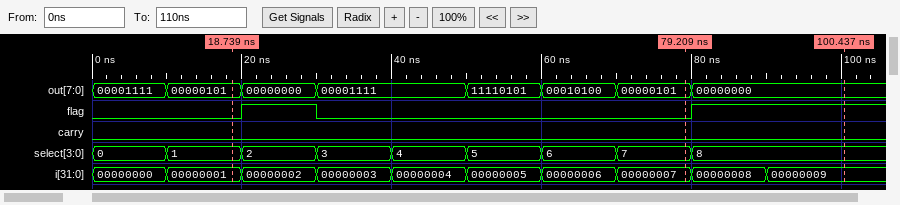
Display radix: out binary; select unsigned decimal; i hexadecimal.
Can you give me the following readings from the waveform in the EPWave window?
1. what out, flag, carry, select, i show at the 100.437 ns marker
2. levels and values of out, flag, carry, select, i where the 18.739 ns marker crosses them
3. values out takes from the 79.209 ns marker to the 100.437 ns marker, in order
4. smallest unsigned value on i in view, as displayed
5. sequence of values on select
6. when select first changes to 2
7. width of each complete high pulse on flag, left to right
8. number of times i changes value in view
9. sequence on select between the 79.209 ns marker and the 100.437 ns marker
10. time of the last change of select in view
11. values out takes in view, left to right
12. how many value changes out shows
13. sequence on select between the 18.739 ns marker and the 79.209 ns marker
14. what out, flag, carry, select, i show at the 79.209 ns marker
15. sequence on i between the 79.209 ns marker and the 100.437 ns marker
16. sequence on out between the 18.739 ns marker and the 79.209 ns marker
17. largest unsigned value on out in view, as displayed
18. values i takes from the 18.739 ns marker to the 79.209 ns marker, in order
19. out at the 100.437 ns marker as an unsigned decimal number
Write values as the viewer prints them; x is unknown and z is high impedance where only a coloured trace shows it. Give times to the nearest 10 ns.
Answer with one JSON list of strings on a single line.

["out=00000000, flag=1, carry=0, select=8, i=00000009", "out=00000101, flag=0, carry=0, select=1, i=00000001", "00000101, 00000000", "00000000", "0, 1, 2, 3, 4, 5, 6, 7, 8", "20 ns", "10 ns", "9", "7, 8", "80 ns", "00001111, 00000101, 00000000, 00001111, 11110101, 00010100, 00000101, 00000000", "7", "1, 2, 3, 4, 5, 6, 7", "out=00000101, flag=0, carry=0, select=7, i=00000007", "00000007, 00000008, 00000009", "00000101, 00000000, 00001111, 11110101, 00010100, 00000101", "11110101", "00000001, 00000002, 00000003, 00000004, 00000005, 00000006, 00000007", "0"]
